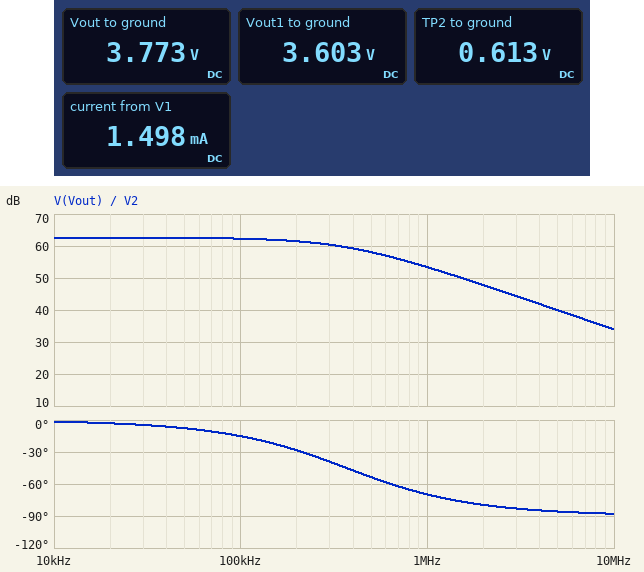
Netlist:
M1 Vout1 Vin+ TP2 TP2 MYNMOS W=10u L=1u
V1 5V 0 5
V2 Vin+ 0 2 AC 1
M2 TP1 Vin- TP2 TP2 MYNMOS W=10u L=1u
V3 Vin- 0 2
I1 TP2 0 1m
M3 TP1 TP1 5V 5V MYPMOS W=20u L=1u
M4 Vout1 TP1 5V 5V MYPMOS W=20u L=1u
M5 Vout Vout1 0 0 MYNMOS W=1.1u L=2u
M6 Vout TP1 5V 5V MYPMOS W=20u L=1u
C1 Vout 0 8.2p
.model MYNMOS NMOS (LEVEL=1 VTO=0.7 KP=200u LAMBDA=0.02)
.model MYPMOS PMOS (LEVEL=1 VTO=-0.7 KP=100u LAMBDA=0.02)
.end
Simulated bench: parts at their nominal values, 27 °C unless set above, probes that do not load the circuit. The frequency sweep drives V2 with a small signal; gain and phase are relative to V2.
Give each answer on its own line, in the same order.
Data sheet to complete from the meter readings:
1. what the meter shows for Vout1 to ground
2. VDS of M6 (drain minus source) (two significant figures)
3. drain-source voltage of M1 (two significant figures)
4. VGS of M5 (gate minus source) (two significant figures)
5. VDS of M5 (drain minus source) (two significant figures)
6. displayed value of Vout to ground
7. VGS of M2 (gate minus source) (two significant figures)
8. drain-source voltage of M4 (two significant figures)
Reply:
3.603 V
-1.2 V
3.0 V
3.6 V
3.8 V
3.773 V
1.4 V
-1.4 V
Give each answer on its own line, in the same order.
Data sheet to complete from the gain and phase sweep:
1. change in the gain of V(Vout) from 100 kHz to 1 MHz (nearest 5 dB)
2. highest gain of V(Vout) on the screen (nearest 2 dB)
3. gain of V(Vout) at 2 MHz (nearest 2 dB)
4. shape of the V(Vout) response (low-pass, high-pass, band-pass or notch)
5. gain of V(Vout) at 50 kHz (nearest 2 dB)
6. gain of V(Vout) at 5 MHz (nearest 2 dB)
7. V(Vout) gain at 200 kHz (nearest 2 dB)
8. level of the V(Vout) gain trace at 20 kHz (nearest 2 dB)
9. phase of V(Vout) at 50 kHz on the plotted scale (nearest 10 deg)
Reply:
-10 dB
62 dB
48 dB
low-pass
62 dB
40 dB
62 dB
62 dB
-10 deg
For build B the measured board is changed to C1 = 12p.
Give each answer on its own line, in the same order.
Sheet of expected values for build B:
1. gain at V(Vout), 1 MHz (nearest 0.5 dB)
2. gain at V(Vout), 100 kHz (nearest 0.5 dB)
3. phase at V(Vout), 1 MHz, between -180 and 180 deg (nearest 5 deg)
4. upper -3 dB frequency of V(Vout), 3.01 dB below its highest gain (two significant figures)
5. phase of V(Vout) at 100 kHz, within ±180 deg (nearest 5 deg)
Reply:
50.5 dB
62.0 dB
-75 deg
250 kHz
-20 deg
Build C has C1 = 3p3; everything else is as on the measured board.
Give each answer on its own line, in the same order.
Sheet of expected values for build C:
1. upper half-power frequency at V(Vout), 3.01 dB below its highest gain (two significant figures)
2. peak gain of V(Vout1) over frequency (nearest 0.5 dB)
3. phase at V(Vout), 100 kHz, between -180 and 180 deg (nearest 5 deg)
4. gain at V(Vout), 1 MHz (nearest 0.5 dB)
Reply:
920 kHz
37.5 dB
-5 deg
59.0 dB
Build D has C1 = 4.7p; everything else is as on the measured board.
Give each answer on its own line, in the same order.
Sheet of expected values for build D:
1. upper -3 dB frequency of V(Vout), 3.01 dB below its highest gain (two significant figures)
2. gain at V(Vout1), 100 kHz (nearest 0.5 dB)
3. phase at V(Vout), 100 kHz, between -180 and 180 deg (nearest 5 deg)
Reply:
640 kHz
37.5 dB
-10 deg
